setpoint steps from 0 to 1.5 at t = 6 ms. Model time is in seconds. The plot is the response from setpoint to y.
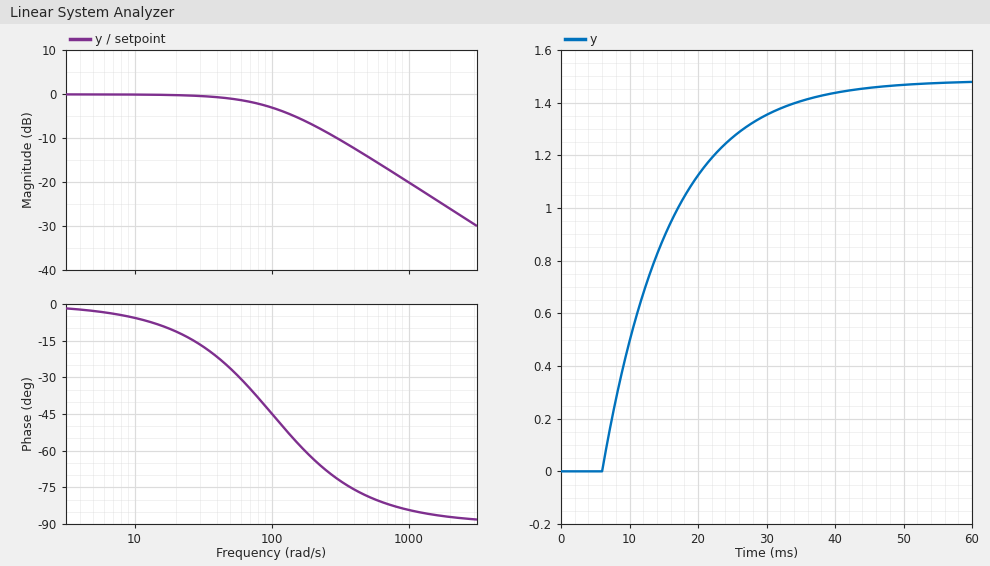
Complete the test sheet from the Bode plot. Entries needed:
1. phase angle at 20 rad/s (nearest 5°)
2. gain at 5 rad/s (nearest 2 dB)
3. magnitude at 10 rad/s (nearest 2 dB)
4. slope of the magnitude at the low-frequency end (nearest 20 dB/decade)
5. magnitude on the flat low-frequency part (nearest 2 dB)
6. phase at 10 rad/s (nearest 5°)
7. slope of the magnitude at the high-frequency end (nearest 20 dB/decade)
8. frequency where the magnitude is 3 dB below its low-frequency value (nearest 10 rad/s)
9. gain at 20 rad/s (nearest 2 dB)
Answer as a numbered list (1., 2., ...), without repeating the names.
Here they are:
1. -10°
2. 0 dB
3. 0 dB
4. 0 dB/decade
5. 0 dB
6. -5°
7. -20 dB/decade
8. 100 rad/s
9. 0 dB
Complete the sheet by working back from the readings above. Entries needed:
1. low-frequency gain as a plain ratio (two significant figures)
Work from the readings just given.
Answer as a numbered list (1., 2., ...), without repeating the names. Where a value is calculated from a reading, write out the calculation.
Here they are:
1. 10^(0 / 20) = 1.0
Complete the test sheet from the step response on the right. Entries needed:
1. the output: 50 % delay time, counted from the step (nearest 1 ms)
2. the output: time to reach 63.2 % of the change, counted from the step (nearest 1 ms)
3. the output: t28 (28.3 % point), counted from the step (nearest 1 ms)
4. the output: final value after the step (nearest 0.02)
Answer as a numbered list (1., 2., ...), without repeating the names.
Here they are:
1. 7 ms
2. 10 ms
3. 3 ms
4. 1.48
